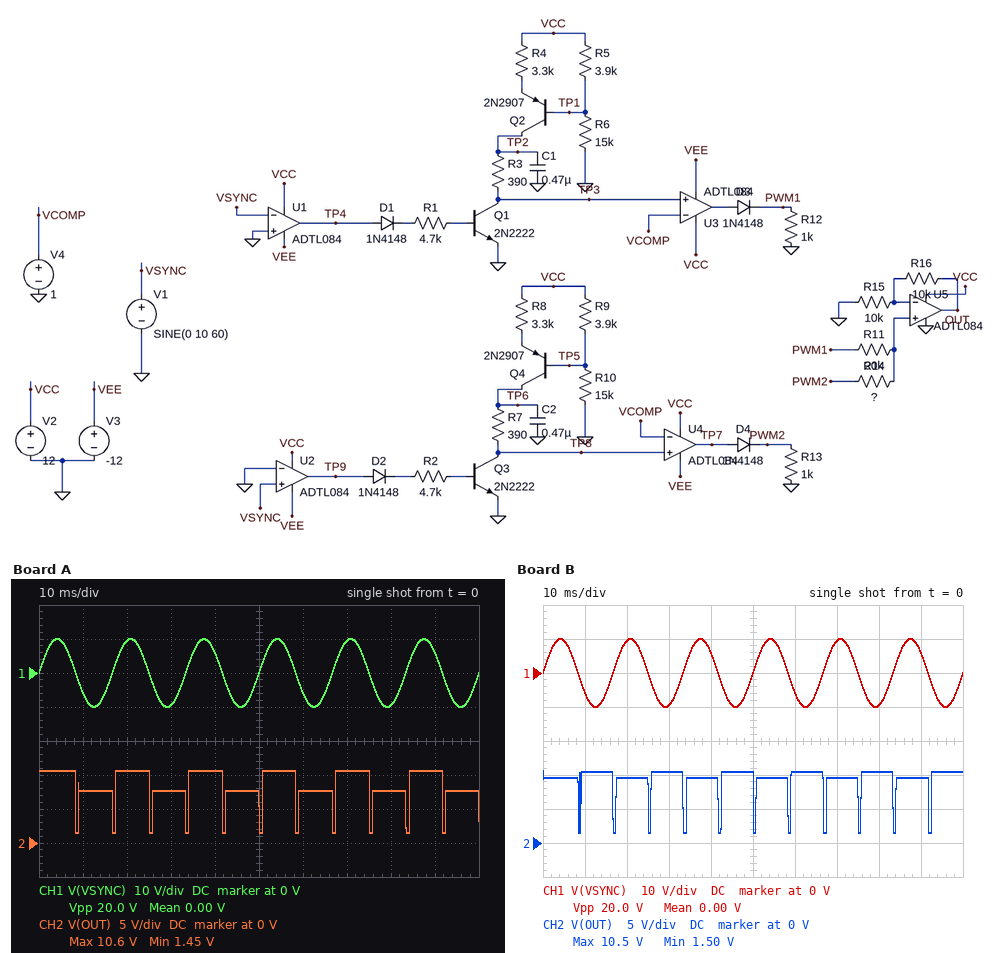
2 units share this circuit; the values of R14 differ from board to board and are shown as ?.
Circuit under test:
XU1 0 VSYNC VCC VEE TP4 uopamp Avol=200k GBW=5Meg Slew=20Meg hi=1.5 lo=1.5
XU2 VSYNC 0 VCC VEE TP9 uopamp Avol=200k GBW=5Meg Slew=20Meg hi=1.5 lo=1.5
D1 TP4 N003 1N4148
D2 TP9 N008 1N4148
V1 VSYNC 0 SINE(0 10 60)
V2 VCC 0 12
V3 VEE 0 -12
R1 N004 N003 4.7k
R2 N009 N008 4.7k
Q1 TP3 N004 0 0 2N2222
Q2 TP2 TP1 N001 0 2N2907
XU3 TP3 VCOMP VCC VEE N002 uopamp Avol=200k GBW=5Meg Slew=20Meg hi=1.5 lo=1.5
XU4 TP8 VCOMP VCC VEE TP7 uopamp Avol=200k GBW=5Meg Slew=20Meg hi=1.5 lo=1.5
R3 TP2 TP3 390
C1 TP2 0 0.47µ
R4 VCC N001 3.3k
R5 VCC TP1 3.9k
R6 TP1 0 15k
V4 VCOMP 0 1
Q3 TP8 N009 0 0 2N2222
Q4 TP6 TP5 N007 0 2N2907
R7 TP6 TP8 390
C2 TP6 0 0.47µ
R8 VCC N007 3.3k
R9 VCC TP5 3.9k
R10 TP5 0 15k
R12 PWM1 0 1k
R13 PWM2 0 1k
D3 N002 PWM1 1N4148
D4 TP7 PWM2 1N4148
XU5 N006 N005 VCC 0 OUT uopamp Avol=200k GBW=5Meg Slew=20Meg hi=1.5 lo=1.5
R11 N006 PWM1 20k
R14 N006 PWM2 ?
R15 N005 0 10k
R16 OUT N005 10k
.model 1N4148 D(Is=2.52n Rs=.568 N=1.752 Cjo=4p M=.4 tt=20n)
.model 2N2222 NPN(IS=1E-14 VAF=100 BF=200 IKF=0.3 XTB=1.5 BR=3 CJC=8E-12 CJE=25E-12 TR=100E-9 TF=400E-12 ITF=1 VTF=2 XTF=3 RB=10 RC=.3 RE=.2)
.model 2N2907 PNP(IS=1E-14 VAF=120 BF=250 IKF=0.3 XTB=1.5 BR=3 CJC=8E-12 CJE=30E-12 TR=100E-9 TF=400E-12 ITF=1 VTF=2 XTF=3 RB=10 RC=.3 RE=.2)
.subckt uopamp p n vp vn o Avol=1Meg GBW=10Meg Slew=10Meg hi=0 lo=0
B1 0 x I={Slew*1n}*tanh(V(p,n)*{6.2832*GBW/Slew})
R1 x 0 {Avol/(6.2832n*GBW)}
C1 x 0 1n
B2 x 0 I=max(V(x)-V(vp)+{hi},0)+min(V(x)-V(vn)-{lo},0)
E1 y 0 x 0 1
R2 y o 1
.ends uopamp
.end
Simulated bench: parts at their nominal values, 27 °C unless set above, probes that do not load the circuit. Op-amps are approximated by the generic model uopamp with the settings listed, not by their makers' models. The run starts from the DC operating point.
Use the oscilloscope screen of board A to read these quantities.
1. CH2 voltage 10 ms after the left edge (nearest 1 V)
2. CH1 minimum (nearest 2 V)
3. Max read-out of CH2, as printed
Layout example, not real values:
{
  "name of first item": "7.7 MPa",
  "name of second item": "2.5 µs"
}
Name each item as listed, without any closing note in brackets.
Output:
{
  "CH2 voltage 10 ms after the left edge": "8 V",
  "CH1 minimum": "-10 V",
  "Max read-out of CH2, as printed": "10.6 V"
}
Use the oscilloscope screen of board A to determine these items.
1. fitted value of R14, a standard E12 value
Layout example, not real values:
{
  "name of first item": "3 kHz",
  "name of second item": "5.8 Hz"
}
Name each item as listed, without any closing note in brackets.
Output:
{
  "fitted value of R14, a standard E12 value": "33 kΩ"
}
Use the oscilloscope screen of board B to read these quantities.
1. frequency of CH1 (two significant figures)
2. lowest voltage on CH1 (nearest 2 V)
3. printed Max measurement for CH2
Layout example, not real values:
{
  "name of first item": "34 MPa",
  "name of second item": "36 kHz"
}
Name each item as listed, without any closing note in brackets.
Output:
{
  "frequency of CH1": "60 Hz",
  "lowest voltage on CH1": "-10 V",
  "printed Max measurement for CH2": "10.5 V"
}
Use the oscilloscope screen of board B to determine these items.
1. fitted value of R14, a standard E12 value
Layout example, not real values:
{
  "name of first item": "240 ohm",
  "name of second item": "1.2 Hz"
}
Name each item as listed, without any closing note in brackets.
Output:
{
  "fitted value of R14, a standard E12 value": "18 kΩ"
}
